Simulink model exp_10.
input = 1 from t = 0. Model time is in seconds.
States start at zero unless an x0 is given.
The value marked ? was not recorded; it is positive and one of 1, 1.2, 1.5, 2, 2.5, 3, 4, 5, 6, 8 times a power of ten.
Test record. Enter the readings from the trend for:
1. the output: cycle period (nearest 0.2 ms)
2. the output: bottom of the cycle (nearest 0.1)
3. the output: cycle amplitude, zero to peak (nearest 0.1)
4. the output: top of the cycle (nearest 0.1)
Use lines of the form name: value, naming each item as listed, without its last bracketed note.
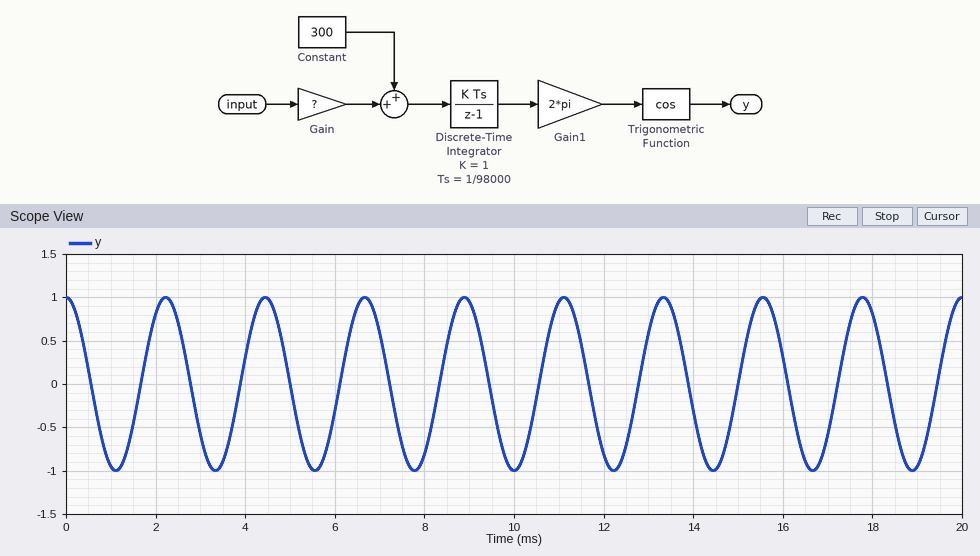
the output: cycle period: 2.2 ms
the output: bottom of the cycle: -1.0
the output: cycle amplitude, zero to peak: 1.0
the output: top of the cycle: 1.0
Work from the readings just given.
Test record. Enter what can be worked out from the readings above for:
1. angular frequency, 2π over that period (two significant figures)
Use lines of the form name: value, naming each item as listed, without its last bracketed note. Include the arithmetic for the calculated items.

angular frequency, 2π over that period: 2π / 2.2 = 2.9 rad/ms
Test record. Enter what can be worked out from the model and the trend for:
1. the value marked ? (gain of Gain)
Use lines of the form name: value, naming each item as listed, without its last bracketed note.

the value marked ?: 150
